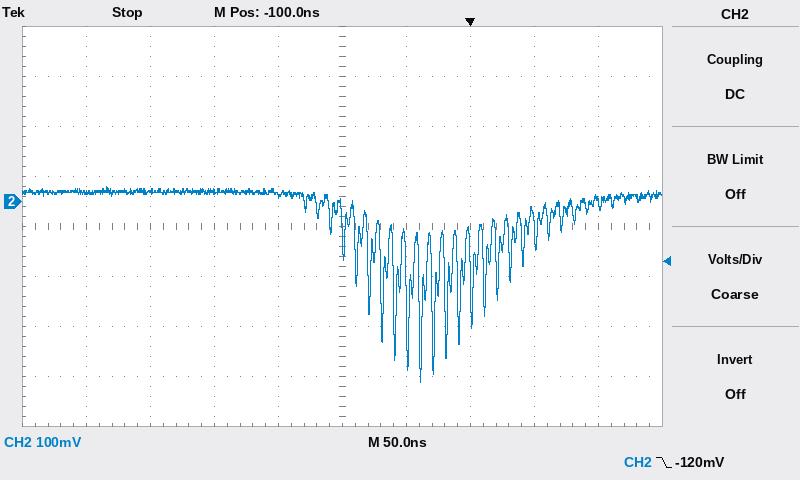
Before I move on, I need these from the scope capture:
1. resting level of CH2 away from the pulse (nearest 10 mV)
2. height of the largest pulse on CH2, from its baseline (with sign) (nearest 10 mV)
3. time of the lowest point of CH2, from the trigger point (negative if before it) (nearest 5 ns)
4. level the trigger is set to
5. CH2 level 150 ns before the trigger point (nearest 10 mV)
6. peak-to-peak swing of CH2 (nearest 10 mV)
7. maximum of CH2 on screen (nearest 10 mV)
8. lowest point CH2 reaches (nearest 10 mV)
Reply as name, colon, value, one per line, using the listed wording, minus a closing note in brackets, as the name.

resting level of CH2 away from the pulse: 20 mV
height of the largest pulse on CH2, from its baseline (with sign): -380 mV
time of the lowest point of CH2, from the trigger point (negative if before it): -40 ns
level the trigger is set to: -120 mV
CH2 level 150 ns before the trigger point: 10 mV
peak-to-peak swing of CH2: 390 mV
maximum of CH2 on screen: 30 mV
lowest point CH2 reaches: -360 mV
